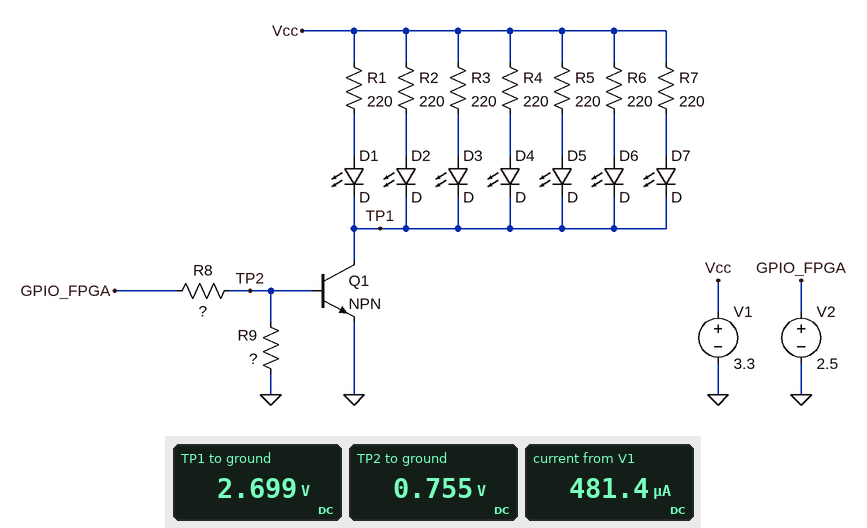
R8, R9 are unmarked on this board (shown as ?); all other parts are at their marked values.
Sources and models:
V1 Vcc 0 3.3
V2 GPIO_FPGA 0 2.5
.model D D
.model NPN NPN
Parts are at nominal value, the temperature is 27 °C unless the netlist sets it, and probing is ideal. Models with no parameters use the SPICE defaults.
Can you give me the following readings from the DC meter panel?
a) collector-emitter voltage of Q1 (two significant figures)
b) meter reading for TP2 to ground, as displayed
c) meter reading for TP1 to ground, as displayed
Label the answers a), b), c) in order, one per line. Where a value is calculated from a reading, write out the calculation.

a) 2.699 V = 2.7 V
b) 0.755 V
c) 2.699 V
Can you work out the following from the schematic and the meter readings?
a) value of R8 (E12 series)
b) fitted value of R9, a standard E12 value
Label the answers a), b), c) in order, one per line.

a) 18 kΩ
b) 8.2 kΩ
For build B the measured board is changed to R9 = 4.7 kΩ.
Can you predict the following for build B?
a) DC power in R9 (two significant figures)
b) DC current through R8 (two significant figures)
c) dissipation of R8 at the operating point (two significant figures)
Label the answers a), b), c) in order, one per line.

a) 57 µW
b) 110 µA
c) 220 µW
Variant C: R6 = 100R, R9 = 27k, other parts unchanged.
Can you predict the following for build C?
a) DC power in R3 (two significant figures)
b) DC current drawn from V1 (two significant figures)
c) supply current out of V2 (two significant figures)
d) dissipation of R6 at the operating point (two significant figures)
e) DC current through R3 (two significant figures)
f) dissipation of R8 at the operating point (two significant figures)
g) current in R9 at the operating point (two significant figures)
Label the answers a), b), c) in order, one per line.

a) 140 µW
b) 6.3 mA
c) 93 µA
d) 240 µW
e) 790 µA
f) 160 µW
g) 30 µA
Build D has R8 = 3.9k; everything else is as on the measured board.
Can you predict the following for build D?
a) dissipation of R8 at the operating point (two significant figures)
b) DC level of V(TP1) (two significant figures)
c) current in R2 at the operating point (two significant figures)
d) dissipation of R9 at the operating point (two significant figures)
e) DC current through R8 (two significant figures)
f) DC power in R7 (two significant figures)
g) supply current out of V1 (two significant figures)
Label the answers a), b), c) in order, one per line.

a) 690 µW
b) 1.6 V
c) 4.5 mA
d) 91 µW
e) 420 µA
f) 4.4 mW
g) 31 mA
